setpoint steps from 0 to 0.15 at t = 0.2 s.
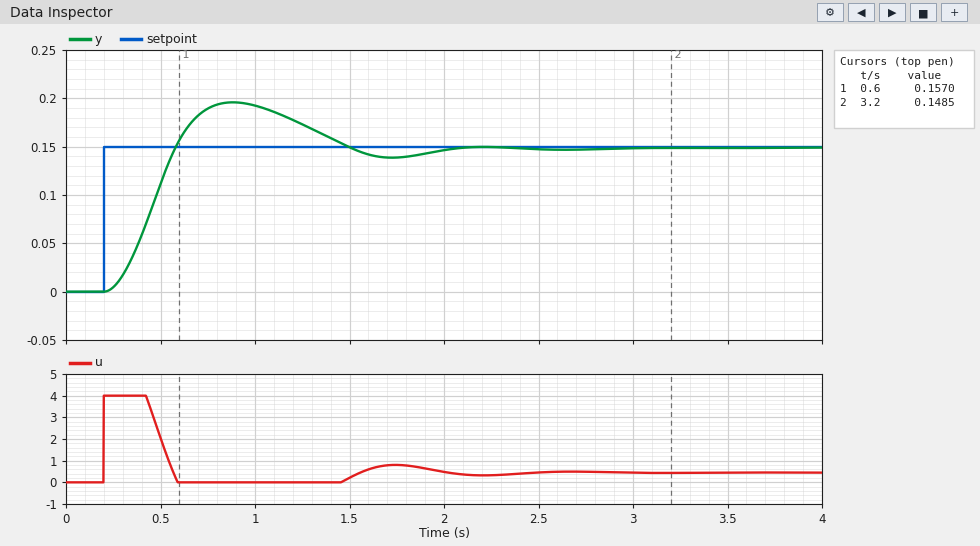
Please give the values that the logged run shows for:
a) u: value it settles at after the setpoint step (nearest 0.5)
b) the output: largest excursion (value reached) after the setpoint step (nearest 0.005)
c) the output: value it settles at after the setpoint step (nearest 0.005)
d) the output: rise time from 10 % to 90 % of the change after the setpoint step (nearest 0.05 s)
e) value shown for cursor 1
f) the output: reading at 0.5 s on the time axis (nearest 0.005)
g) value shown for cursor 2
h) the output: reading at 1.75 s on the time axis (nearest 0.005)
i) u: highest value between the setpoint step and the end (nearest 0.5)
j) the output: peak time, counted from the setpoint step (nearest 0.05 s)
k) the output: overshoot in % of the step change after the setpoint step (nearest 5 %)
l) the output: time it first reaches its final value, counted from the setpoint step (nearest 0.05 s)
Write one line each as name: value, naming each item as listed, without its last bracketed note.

u: value it settles at after the setpoint step: 0.5
the output: largest excursion (value reached) after the setpoint step: 0.195
the output: value it settles at after the setpoint step: 0.150
the output: rise time from 10 % to 90 % of the change after the setpoint step: 0.25 s
value shown for cursor 1: 0.1570
the output: reading at 0.5 s on the time axis: 0.110
value shown for cursor 2: 0.1485
the output: reading at 1.75 s on the time axis: 0.140
u: highest value between the setpoint step and the end: 4.0
the output: peak time, counted from the setpoint step: 0.70 s
the output: overshoot in % of the step change after the setpoint step: 30 %
the output: time it first reaches its final value, counted from the setpoint step: 0.40 s
